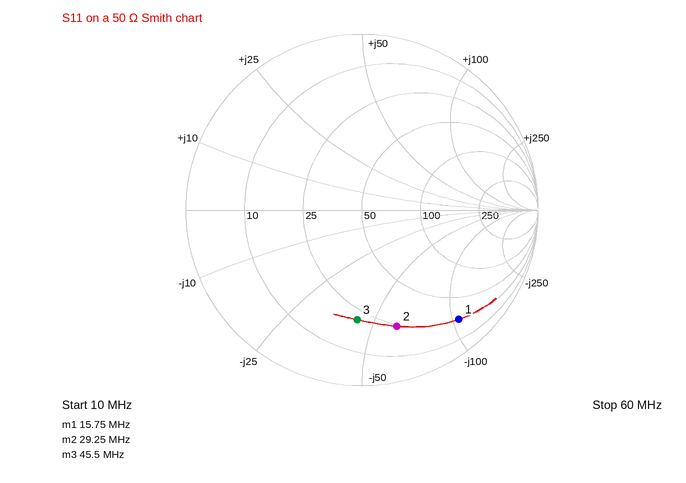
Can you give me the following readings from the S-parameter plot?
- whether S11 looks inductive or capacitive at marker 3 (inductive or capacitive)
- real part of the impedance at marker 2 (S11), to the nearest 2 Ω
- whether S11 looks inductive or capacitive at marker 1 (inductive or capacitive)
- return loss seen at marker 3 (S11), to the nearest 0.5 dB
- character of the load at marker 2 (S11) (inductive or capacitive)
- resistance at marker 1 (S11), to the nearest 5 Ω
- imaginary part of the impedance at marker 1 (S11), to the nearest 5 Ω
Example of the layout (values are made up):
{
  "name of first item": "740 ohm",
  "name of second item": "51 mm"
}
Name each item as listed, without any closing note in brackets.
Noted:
{
  "whether S11 looks inductive or capacitive at marker 3": "capacitive",
  "real part of the impedance at marker 2 (S11), to the nearest 2 Ω": "24 Ω",
  "whether S11 looks inductive or capacitive at marker 1": "capacitive",
  "return loss seen at marker 3 (S11), to the nearest 0.5 dB": "4.0 dB",
  "character of the load at marker 2 (S11)": "capacitive",
  "resistance at marker 1 (S11), to the nearest 5 Ω": "25 Ω",
  "imaginary part of the impedance at marker 1 (S11), to the nearest 5 Ω": "-105 Ω"
}
